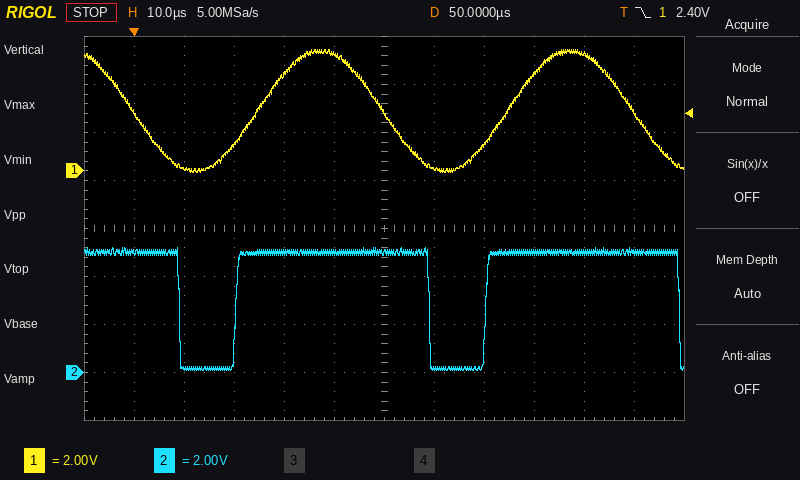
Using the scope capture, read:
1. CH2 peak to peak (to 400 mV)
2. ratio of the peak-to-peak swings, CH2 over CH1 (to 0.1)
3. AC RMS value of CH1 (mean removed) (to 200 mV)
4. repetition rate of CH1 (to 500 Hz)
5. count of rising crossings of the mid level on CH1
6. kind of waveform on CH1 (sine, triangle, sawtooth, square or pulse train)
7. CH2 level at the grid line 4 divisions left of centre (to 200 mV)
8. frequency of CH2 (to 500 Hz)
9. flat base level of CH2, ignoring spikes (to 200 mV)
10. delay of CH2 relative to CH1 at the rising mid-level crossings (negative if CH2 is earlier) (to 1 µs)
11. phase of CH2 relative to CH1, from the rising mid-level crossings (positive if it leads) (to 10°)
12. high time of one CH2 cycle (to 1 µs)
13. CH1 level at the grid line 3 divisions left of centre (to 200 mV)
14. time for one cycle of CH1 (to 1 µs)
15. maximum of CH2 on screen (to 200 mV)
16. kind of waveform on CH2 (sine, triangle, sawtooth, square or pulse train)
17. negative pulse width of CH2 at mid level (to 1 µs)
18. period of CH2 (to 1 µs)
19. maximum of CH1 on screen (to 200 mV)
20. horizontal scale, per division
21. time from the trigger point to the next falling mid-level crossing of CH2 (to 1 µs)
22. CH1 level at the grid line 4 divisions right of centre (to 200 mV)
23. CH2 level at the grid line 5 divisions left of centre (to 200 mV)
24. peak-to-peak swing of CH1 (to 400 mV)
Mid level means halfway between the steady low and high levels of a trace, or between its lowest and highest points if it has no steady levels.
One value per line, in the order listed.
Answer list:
5.2 V
1.0
1.8 V
20.0 kHz
2
sine
200 mV
20.0 kHz
200 mV
-4 µs
+30°
39 µs
1.0 V
50 µs
5.2 V
pulse train
11 µs
50 µs
5.0 V
10 µs
9 µs
4.8 V
5.0 V
5.2 V
